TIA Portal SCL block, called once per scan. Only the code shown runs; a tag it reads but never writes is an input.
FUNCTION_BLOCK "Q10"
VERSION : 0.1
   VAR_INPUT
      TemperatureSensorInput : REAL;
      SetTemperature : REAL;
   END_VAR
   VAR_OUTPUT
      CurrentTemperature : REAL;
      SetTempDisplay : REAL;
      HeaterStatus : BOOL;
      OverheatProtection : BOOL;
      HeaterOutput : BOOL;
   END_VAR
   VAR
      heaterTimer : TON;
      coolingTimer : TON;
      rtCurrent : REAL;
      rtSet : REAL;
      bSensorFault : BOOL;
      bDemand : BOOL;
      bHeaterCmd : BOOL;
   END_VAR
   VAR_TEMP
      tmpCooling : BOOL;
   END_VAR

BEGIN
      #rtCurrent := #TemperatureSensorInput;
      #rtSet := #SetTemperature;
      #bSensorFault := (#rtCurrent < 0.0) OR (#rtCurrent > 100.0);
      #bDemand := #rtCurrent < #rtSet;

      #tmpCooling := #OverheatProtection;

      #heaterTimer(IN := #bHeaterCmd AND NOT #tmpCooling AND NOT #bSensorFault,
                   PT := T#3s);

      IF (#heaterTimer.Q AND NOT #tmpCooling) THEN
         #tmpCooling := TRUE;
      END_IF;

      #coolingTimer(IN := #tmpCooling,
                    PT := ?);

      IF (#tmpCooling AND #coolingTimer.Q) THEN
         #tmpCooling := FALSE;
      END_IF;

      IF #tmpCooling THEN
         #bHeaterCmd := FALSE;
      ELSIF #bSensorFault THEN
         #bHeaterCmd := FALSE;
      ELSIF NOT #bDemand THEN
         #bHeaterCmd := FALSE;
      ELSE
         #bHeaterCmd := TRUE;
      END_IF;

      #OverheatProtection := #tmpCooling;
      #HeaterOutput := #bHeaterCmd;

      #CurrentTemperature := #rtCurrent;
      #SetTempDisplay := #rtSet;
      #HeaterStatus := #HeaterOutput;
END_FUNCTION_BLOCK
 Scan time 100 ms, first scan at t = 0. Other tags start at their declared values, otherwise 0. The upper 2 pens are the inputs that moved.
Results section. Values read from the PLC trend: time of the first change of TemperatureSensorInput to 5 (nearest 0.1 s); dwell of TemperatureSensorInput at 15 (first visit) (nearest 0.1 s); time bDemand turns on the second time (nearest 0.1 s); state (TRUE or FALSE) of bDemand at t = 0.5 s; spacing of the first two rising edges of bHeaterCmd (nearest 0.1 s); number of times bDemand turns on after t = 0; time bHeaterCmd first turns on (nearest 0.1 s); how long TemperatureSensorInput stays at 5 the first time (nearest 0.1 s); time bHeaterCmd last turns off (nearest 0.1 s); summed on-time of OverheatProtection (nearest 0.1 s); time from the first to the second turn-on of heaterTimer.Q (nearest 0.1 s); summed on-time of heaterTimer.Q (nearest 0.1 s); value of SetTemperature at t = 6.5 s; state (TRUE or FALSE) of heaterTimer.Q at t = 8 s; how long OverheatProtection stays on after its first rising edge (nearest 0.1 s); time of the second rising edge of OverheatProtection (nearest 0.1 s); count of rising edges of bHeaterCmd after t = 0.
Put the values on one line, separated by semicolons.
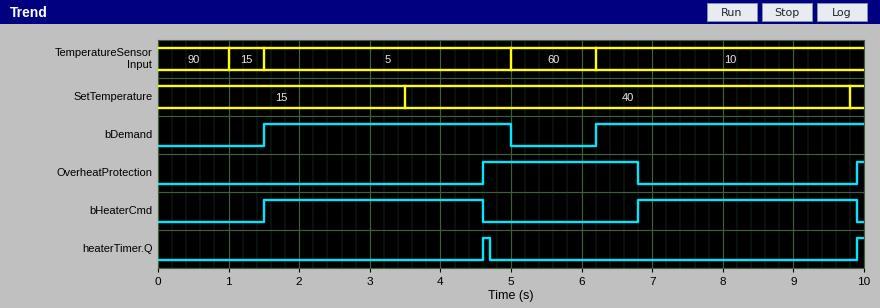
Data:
1.5 s; 0.5 s; 6.2 s; FALSE; 5.3 s; 2; 1.5 s; 3.5 s; 9.9 s; 2.3 s; 5.3 s; 0.2 s; 40; FALSE; 2.2 s; 9.9 s; 2
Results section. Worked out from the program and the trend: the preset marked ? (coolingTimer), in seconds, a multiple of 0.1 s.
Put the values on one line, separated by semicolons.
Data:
2.2 s
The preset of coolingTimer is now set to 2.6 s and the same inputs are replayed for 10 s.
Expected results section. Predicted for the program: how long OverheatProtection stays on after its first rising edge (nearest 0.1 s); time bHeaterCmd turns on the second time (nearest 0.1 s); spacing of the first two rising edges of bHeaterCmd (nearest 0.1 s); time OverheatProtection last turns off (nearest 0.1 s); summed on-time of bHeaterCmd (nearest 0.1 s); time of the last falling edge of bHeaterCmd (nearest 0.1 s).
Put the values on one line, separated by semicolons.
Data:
2.6 s; 7.2 s; 5.7 s; 7.2 s; 5.9 s; 4.6 s
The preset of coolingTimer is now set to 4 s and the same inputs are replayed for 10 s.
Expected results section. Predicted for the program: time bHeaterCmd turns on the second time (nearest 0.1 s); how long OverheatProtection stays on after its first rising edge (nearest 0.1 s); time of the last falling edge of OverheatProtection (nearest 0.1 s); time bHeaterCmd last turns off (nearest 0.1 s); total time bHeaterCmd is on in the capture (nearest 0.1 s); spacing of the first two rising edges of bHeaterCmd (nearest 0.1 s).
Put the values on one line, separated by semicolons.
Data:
8.6 s; 4.0 s; 8.6 s; 4.6 s; 4.5 s; 7.1 s
